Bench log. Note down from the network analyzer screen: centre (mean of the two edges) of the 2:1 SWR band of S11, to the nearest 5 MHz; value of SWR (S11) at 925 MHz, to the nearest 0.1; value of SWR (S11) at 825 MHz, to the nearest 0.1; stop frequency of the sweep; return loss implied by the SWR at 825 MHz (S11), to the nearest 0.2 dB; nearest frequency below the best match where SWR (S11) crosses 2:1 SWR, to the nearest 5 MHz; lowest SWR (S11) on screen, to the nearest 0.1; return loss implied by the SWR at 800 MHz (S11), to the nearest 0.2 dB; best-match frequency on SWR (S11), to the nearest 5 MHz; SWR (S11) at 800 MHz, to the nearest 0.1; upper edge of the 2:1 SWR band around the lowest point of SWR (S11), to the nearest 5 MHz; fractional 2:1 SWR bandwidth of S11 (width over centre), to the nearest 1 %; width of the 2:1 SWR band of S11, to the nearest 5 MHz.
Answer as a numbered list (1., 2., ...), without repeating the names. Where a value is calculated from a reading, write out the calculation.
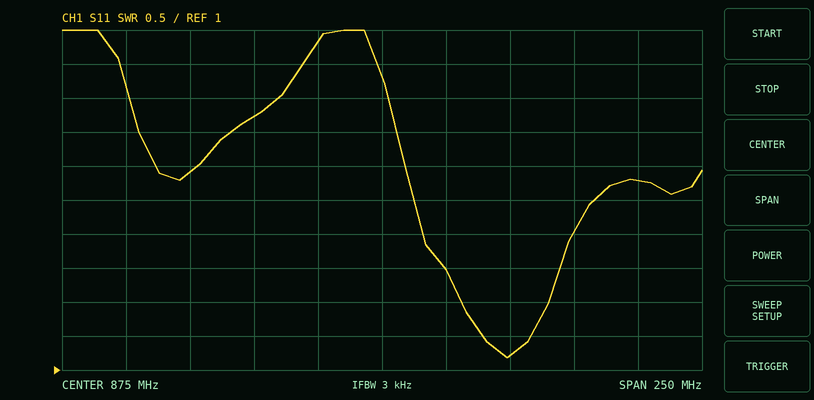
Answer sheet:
1. 925 MHz
2. 1.2
3. 4.7
4. 1 GHz
5. −20 log10((4.7 − 1)/(4.7 + 1)) ≈ 3.8 dB
6. 905 MHz
7. 1.2
8. −20 log10((3.9 − 1)/(3.9 + 1)) ≈ 4.6 dB
9. 925 MHz
10. 3.9
11. 940 MHz
12. 35 MHz / 922.5 MHz ≈ 4 %
13. 940 MHz − 905 MHz = 35 MHz
